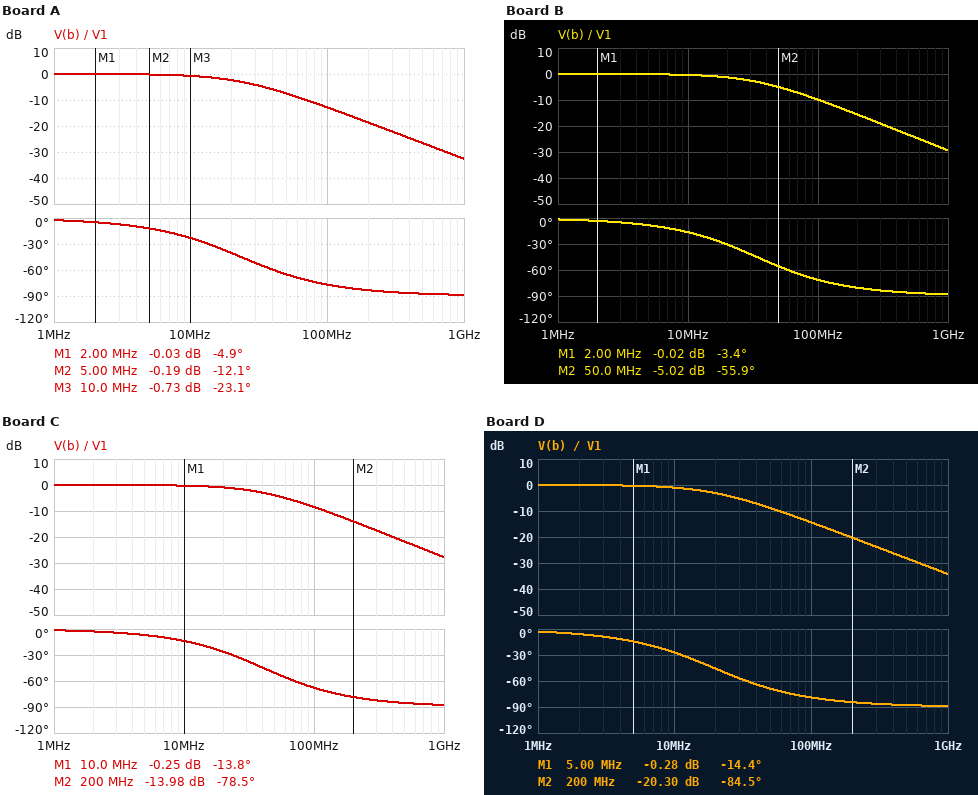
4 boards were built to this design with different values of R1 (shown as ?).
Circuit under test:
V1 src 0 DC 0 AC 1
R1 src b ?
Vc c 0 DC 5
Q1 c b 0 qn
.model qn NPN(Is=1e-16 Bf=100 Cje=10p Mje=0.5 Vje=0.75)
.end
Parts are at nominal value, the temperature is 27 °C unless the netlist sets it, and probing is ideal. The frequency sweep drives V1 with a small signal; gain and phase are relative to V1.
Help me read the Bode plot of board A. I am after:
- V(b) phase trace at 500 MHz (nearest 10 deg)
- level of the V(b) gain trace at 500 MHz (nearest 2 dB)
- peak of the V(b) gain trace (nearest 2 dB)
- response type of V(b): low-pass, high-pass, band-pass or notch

-90 deg
-26 dB
0 dB
low-pass
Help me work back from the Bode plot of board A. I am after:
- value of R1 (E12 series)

680 Ω
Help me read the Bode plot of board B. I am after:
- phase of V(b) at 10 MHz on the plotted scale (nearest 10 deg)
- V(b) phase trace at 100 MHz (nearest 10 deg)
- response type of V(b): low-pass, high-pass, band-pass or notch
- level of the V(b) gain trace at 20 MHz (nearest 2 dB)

-20 deg
-70 deg
low-pass
-2 dB
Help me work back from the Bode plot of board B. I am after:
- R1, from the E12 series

470 Ω
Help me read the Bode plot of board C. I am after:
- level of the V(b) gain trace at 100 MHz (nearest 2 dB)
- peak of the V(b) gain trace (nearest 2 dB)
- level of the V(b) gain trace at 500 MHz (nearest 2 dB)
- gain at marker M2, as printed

-8 dB
0 dB
-22 dB
-13.98 dB
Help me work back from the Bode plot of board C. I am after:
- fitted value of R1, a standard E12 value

390 Ω
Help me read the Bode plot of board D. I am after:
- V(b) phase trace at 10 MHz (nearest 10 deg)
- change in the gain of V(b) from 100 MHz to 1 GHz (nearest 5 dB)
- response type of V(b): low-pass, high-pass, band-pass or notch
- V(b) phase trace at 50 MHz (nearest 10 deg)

-30 deg
-20 dB
low-pass
-70 deg
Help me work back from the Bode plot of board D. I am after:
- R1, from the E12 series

820 Ω
